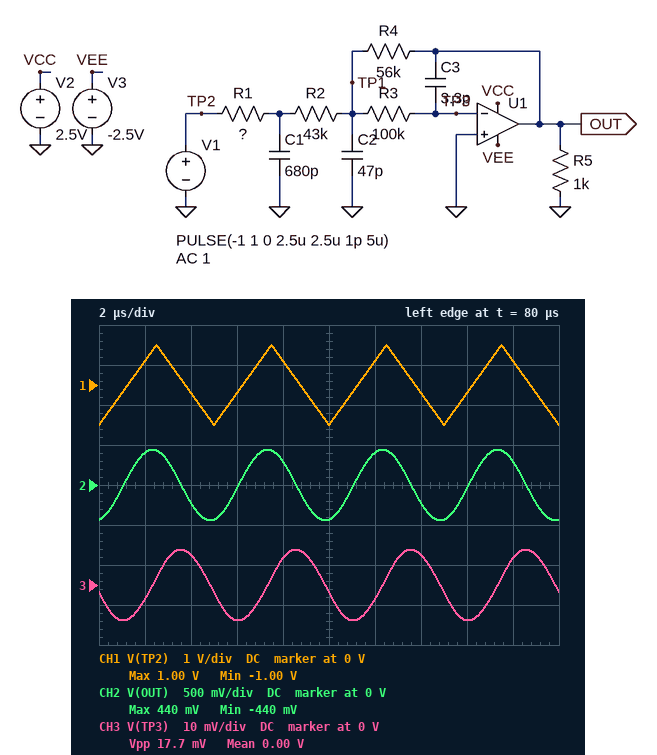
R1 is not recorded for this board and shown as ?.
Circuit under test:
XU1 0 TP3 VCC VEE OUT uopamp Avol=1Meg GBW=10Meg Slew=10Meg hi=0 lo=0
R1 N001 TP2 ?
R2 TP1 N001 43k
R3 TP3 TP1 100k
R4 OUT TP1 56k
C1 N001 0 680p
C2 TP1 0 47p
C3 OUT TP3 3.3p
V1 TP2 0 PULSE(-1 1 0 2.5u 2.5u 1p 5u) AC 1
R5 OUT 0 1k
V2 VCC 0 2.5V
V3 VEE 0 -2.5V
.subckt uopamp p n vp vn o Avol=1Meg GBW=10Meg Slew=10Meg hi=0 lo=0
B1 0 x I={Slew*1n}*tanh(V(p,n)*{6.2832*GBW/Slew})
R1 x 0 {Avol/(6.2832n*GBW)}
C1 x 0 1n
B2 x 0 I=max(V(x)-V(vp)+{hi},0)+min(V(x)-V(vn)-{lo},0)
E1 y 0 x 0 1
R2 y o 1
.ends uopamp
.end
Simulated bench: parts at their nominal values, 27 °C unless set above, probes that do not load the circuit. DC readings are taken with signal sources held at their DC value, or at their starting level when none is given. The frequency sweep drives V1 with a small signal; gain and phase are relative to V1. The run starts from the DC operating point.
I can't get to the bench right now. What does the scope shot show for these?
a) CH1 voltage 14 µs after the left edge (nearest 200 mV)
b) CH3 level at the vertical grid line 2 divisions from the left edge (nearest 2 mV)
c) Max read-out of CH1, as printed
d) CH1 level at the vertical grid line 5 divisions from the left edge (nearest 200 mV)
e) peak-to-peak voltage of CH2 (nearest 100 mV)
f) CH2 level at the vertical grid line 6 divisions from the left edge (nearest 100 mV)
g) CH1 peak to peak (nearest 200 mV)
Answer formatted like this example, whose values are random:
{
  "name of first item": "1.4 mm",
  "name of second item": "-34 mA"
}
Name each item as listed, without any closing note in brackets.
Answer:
{
  "CH1 voltage 14 µs after the left edge": "-200 mV",
  "CH3 level at the vertical grid line 2 divisions from the left edge": "8 mV",
  "Max read-out of CH1, as printed": "1.00 V",
  "CH1 level at the vertical grid line 5 divisions from the left edge": "-1.0 V",
  "peak-to-peak voltage of CH2": "900 mV",
  "CH2 level at the vertical grid line 6 divisions from the left edge": "400 mV",
  "CH1 peak to peak": "2.0 V"
}
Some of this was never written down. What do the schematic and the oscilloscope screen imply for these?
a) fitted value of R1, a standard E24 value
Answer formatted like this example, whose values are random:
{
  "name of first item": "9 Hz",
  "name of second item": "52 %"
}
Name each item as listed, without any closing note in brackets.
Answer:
{
  "fitted value of R1, a standard E24 value": "1.8 kΩ"
}
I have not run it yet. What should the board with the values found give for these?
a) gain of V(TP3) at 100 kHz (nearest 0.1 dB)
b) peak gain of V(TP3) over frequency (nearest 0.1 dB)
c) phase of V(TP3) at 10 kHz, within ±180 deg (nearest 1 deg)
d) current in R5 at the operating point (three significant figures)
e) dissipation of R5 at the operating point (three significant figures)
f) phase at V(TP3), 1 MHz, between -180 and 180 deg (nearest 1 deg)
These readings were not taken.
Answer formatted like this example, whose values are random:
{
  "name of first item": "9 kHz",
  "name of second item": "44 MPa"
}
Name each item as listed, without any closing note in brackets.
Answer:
{
  "gain of V(TP3) at 100 kHz": "-38.8 dB",
  "peak gain of V(TP3) over frequency": "-37.3 dB",
  "phase of V(TP3) at 10 kHz, within ±180 deg": "82 deg",
  "current in R5 at the operating point": "1.25 mA",
  "dissipation of R5 at the operating point": "1.56 mW",
  "phase at V(TP3), 1 MHz, between -180 and 180 deg": "-168 deg"
}
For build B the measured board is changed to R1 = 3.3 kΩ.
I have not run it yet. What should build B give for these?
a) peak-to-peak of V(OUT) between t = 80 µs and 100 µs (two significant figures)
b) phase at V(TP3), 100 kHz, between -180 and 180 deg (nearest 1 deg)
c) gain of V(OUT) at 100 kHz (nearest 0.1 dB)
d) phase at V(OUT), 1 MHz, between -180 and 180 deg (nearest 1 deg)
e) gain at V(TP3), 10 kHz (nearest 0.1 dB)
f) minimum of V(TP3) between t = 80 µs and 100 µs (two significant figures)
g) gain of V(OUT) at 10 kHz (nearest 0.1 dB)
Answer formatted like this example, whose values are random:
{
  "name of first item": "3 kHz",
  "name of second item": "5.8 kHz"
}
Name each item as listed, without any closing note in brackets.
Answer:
{
  "peak-to-peak of V(OUT) between t = 80 µs and 100 µs": "540 mV",
  "phase at V(TP3), 100 kHz, between -180 and 180 deg": "-7 deg",
  "gain of V(OUT) at 100 kHz": "-1.5 dB",
  "phase at V(OUT), 1 MHz, between -180 and 180 deg": "-81 deg",
  "gain at V(TP3), 10 kHz": "-58.4 dB",
  "minimum of V(TP3) between t = 80 µs and 100 µs": "-5.4 mV",
  "gain of V(OUT) at 10 kHz": "1.6 dB"
}
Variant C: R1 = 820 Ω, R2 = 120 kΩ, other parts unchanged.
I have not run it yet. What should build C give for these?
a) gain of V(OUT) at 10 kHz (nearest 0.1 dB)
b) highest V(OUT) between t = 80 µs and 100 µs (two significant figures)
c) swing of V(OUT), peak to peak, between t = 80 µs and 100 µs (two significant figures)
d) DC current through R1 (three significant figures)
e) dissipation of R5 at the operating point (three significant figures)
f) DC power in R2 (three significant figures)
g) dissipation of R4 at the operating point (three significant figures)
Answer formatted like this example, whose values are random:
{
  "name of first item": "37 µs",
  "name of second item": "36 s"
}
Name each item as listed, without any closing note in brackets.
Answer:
{
  "gain of V(OUT) at 10 kHz": "-6.7 dB",
  "highest V(OUT) between t = 80 µs and 100 µs": "320 mV",
  "swing of V(OUT), peak to peak, between t = 80 µs and 100 µs": "640 mV",
  "DC current through R1": "8.28 µA",
  "dissipation of R5 at the operating point": "215 µW",
  "DC power in R2": "8.22 µW",
  "dissipation of R4 at the operating point": "3.84 µW"
}
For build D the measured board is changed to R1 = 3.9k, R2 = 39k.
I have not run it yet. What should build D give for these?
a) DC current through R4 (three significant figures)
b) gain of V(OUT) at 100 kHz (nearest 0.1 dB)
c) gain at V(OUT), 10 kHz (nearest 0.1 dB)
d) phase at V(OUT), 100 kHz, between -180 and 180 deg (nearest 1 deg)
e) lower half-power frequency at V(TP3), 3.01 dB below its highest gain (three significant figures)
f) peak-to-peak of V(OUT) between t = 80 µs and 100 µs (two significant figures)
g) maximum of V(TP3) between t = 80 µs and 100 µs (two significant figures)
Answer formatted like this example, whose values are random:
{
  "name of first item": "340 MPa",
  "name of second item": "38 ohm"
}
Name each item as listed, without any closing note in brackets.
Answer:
{
  "DC current through R4": "23.3 µA",
  "gain of V(OUT) at 100 kHz": "-1.8 dB",
  "gain at V(OUT), 10 kHz": "2.2 dB",
  "phase at V(OUT), 100 kHz, between -180 and 180 deg": "78 deg",
  "lower half-power frequency at V(TP3), 3.01 dB below its highest gain": "57.9 kHz",
  "peak-to-peak of V(OUT) between t = 80 µs and 100 µs": "490 mV",
  "maximum of V(TP3) between t = 80 µs and 100 µs": "4.9 mV"
}
